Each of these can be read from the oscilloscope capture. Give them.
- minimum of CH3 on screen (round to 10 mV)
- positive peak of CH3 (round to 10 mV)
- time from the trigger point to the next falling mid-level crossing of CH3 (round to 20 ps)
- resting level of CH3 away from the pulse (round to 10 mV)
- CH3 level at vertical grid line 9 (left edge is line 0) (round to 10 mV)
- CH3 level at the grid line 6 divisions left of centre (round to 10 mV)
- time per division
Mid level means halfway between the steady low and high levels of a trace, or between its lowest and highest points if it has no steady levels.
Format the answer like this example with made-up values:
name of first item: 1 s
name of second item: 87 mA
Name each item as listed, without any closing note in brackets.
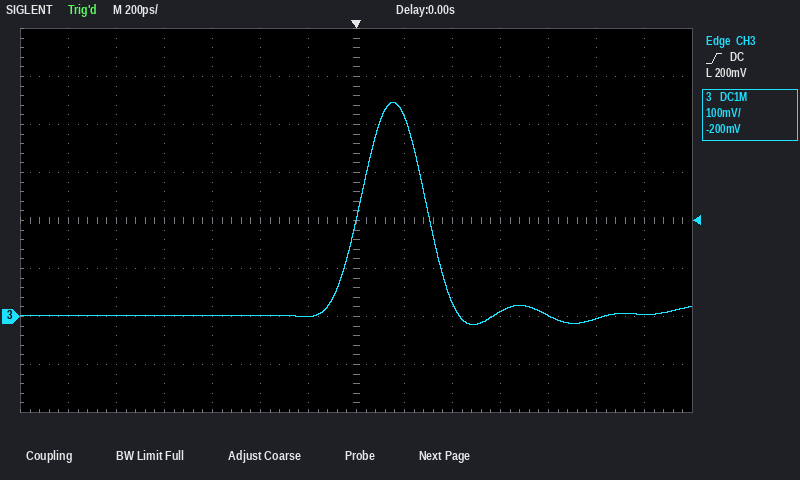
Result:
minimum of CH3 on screen: -20 mV
positive peak of CH3: 450 mV
time from the trigger point to the next falling mid-level crossing of CH3: 300 ps
resting level of CH3 away from the pulse: 0 mV
CH3 level at vertical grid line 9 (left edge is line 0): 30 mV
CH3 level at the grid line 6 divisions left of centre: 0 mV
time per division: 200 ps
